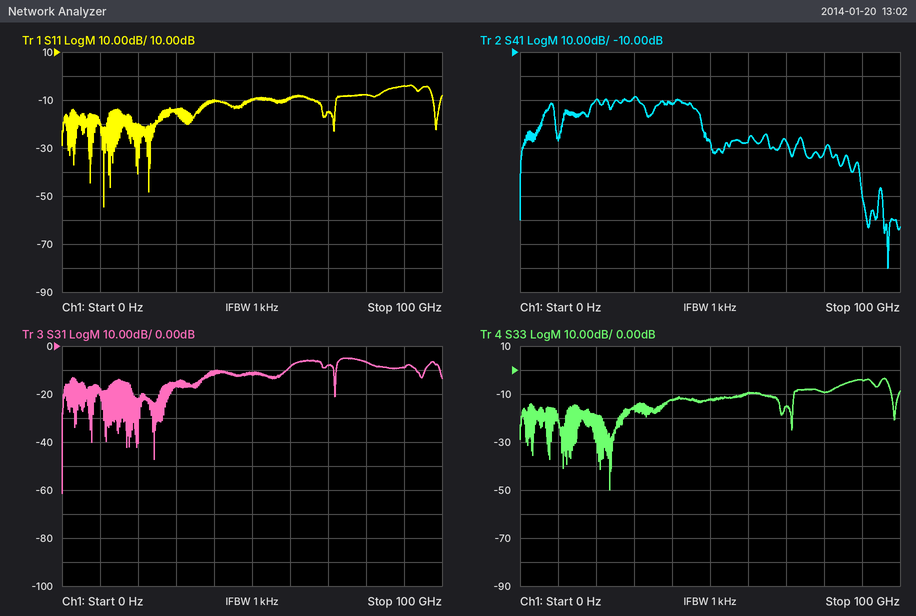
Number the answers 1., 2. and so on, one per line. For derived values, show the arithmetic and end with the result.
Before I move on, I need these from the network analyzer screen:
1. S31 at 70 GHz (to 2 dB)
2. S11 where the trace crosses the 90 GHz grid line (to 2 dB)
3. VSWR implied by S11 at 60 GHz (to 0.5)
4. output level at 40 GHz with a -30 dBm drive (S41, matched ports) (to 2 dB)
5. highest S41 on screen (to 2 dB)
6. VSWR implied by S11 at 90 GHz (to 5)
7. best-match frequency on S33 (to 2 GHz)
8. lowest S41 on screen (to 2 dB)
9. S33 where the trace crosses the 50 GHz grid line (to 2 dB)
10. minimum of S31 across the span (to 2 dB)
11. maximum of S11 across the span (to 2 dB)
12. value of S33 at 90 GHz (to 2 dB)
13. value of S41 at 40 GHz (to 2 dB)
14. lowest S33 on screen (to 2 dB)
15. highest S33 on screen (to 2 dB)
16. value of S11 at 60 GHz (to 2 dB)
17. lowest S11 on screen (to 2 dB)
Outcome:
1. -8 dB
2. -4 dB
3. |Γ| = 10^(-10/20) = 0.3162; VSWR = (1 + 0.3162)/(1 − 0.3162) ≈ 1.92, so 2.0 to the nearest 0.5
4. -30 dBm + (-32 dB) = -62 dBm
5. -28 dB
6. |Γ| = 10^(-4/20) = 0.6310; VSWR = (1 + 0.6310)/(1 − 0.6310) ≈ 4.42, so 5 to the nearest 5
7. 24 GHz
8. -100 dB
9. -12 dB
10. -62 dB
11. -4 dB
12. -4 dB
13. -32 dB
14. -50 dB
15. -4 dB
16. -10 dB
17. -54 dB
